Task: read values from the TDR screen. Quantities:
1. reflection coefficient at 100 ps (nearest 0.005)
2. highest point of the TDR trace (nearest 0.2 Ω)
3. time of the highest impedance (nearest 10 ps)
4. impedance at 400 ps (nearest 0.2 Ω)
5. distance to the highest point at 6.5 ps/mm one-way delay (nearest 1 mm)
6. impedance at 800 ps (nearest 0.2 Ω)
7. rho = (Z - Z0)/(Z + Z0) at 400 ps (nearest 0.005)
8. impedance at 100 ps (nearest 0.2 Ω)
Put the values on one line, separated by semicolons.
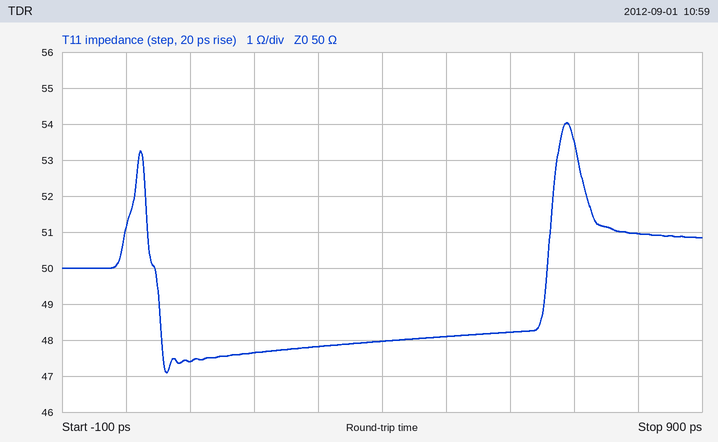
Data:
-0.025; 54.0 Ω; 690 ps; 48.0 Ω; 53 mm; 51.0 Ω; -0.020; 47.4 Ω
